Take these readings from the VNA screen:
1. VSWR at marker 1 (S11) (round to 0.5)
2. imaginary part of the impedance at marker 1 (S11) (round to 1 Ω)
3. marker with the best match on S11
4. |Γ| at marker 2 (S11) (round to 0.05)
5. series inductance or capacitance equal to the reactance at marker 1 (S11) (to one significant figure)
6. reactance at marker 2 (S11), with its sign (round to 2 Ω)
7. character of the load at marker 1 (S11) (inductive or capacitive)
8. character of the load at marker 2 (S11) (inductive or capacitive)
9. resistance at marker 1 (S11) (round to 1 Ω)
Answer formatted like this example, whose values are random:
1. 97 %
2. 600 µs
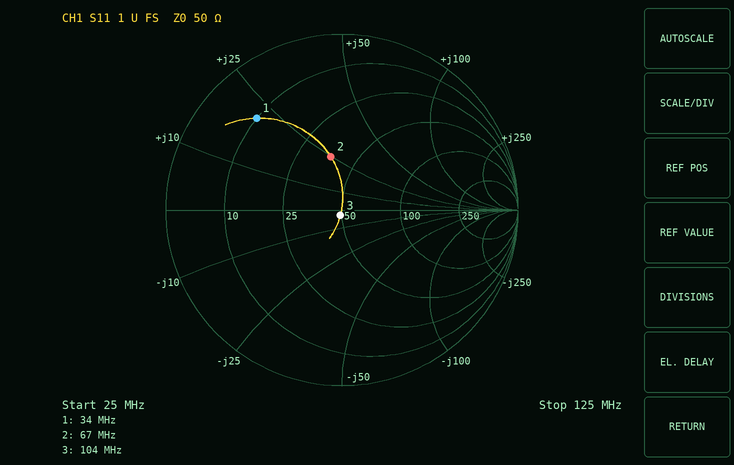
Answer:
1. 6.0
2. +21 Ω
3. marker 3
4. 0.30
5. 100 nH
6. +24 Ω
7. inductive
8. inductive
9. 10 Ω
